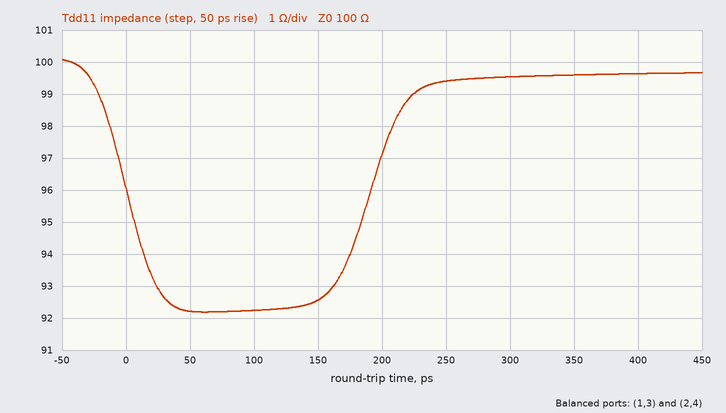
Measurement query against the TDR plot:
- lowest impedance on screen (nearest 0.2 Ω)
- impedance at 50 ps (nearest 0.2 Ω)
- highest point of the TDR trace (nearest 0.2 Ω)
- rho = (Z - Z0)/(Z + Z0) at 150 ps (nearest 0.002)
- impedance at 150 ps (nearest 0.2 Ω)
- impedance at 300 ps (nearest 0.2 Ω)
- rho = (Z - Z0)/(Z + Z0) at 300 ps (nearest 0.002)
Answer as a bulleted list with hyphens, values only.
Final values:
- 92.2 Ω
- 92.2 Ω
- 100.0 Ω
- -0.038
- 92.6 Ω
- 99.6 Ω
- -0.002
